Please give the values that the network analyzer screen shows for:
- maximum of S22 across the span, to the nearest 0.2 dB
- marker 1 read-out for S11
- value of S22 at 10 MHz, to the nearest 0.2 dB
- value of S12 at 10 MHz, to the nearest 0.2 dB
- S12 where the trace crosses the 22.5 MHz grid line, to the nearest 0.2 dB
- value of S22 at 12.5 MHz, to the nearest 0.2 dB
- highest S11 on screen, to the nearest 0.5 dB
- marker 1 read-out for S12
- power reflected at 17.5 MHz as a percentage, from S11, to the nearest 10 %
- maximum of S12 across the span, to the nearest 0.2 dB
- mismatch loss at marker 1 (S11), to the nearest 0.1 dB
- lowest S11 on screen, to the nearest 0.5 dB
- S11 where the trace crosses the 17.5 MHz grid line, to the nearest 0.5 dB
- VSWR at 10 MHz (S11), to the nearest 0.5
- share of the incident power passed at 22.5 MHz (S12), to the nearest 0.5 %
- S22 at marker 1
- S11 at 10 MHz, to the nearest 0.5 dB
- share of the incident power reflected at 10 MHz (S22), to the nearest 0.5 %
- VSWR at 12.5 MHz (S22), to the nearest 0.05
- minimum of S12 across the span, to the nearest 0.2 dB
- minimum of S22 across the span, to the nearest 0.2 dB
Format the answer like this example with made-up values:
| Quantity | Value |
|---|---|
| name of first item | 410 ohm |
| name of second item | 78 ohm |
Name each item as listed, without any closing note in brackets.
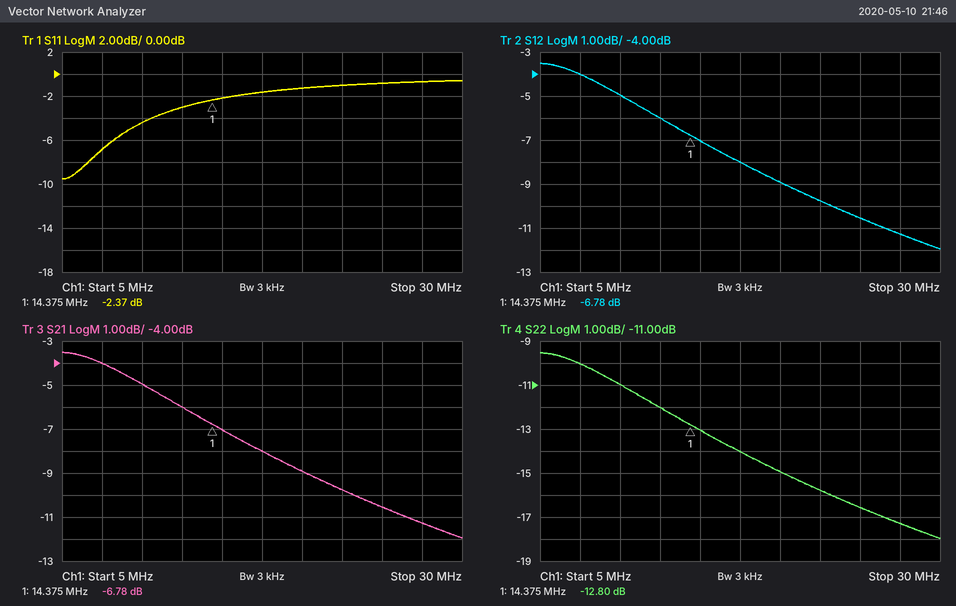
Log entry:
| Quantity | Value |
|---|---|
| maximum of S22 across the span, to the nearest 0.2 dB | -9.6 dB |
| marker 1 read-out for S11 | -2.37 dB |
| value of S22 at 10 MHz, to the nearest 0.2 dB | -11.0 dB |
| value of S12 at 10 MHz, to the nearest 0.2 dB | -5.0 dB |
| S12 where the trace crosses the 22.5 MHz grid line, to the nearest 0.2 dB | -9.8 dB |
| value of S22 at 12.5 MHz, to the nearest 0.2 dB | -12.0 dB |
| highest S11 on screen, to the nearest 0.5 dB | -0.5 dB |
| marker 1 read-out for S12 | -6.78 dB |
| power reflected at 17.5 MHz as a percentage, from S11, to the nearest 10 % | 70 % |
| maximum of S12 across the span, to the nearest 0.2 dB | -3.6 dB |
| mismatch loss at marker 1 (S11), to the nearest 0.1 dB | 3.8 dB |
| lowest S11 on screen, to the nearest 0.5 dB | -9.5 dB |
| S11 where the trace crosses the 17.5 MHz grid line, to the nearest 0.5 dB | -1.5 dB |
| VSWR at 10 MHz (S11), to the nearest 0.5 | 4.0 |
| share of the incident power passed at 22.5 MHz (S12), to the nearest 0.5 % | 10.5 % |
| S22 at marker 1 | -12.80 dB |
| S11 at 10 MHz, to the nearest 0.5 dB | -4.5 dB |
| share of the incident power reflected at 10 MHz (S22), to the nearest 0.5 % | 8.0 % |
| VSWR at 12.5 MHz (S22), to the nearest 0.05 | 1.65 |
| minimum of S12 across the span, to the nearest 0.2 dB | -12.0 dB |
| minimum of S22 across the span, to the nearest 0.2 dB | -18.0 dB |
